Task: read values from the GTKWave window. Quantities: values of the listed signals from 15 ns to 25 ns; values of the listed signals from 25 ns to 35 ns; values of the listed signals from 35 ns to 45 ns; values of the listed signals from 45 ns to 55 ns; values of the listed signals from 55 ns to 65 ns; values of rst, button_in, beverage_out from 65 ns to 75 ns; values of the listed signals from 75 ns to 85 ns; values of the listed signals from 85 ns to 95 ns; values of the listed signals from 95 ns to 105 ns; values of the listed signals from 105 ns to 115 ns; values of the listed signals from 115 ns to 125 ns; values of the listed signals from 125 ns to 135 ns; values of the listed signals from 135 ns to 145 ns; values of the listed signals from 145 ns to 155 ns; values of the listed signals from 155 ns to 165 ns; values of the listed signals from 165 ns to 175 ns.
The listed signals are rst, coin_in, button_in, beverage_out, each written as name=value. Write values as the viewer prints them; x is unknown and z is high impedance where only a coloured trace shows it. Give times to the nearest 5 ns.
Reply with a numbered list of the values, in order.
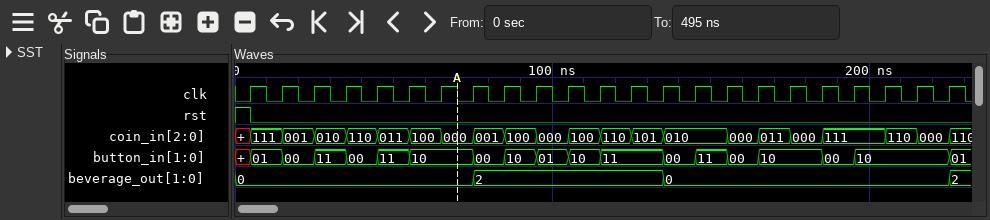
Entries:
1. rst=0, coin_in=001, button_in=00, beverage_out=0
2. rst=0, coin_in=010, button_in=11, beverage_out=0
3. rst=0, coin_in=110, button_in=00, beverage_out=0
4. rst=0, coin_in=011, button_in=11, beverage_out=0
5. rst=0, coin_in=100, button_in=10, beverage_out=0
6. rst=0, button_in=10, beverage_out=0
7. rst=0, coin_in=001, button_in=00, beverage_out=2
8. rst=0, coin_in=100, button_in=10, beverage_out=2
9. rst=0, coin_in=000, button_in=01, beverage_out=2
10. rst=0, coin_in=100, button_in=10, beverage_out=2
11. rst=0, coin_in=110, button_in=11, beverage_out=2
12. rst=0, coin_in=101, button_in=11, beverage_out=2
13. rst=0, coin_in=010, button_in=00, beverage_out=0
14. rst=0, coin_in=010, button_in=11, beverage_out=0
15. rst=0, coin_in=000, button_in=00, beverage_out=0
16. rst=0, coin_in=011, button_in=10, beverage_out=0
